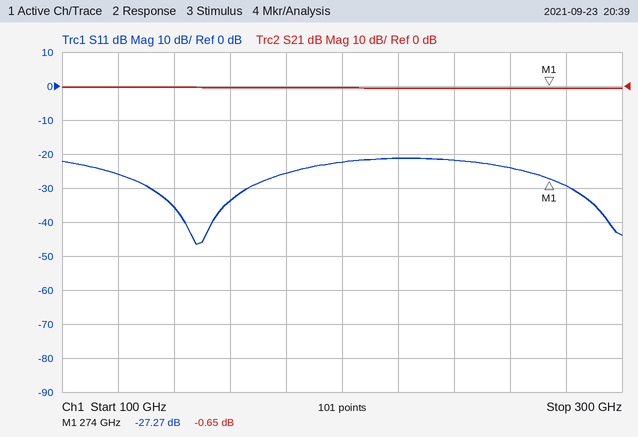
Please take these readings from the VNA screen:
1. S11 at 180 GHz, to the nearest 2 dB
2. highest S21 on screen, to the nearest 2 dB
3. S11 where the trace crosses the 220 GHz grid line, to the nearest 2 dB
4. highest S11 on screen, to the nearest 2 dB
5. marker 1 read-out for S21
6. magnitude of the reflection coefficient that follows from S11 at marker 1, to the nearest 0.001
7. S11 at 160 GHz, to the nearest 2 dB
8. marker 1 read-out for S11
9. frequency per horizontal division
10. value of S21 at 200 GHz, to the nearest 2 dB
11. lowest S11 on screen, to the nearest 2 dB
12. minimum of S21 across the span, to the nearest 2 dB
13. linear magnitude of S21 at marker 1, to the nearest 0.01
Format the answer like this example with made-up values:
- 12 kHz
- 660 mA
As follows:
- -26 dB
- 0 dB
- -22 dB
- -22 dB
- -0.65 dB
- 0.043
- -34 dB
- -27.27 dB
- 20 GHz
- 0 dB
- -46 dB
- 0 dB
- 0.93
